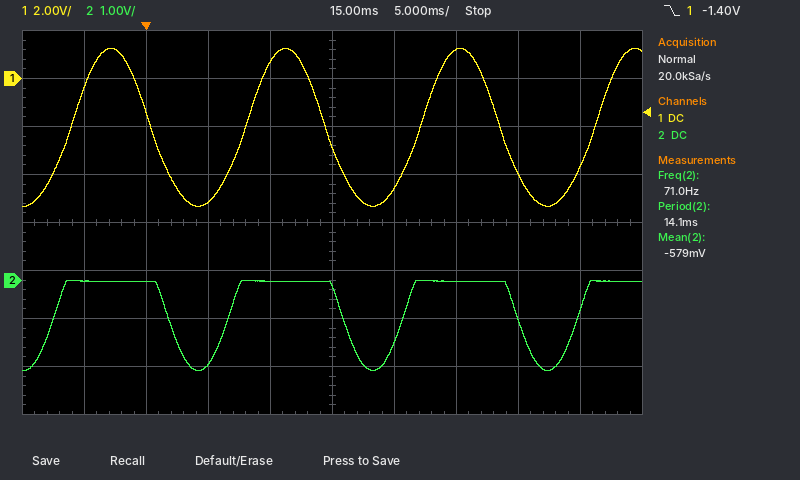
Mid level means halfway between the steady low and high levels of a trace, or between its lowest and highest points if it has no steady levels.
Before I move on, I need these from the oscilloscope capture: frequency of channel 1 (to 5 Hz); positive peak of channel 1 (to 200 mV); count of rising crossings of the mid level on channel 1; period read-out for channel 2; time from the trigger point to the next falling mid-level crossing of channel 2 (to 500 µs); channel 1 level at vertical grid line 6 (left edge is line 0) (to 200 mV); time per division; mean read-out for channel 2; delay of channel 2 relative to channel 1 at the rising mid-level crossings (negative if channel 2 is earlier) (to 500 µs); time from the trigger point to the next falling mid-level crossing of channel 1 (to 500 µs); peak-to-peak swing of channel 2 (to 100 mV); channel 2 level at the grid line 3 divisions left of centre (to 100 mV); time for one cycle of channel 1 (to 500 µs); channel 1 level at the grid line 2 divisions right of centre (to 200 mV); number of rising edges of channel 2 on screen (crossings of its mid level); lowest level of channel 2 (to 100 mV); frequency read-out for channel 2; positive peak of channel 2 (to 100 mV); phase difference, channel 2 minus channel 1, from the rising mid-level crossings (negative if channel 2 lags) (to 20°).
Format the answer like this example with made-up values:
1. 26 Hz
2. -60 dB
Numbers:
1. 70 Hz
2. 1.2 V
3. 4
4. 14.1 ms
5. 2.0 ms
6. -4.6 V
7. 5 ms
8. -579 mV
9. -1.5 ms
10. 500 µs
11. 1.9 V
12. 0.0 V
13. 14.0 ms
14. 1.2 V
15. 4
16. -1.9 V
17. 71.0 Hz
18. 0.0 V
19. +40°
